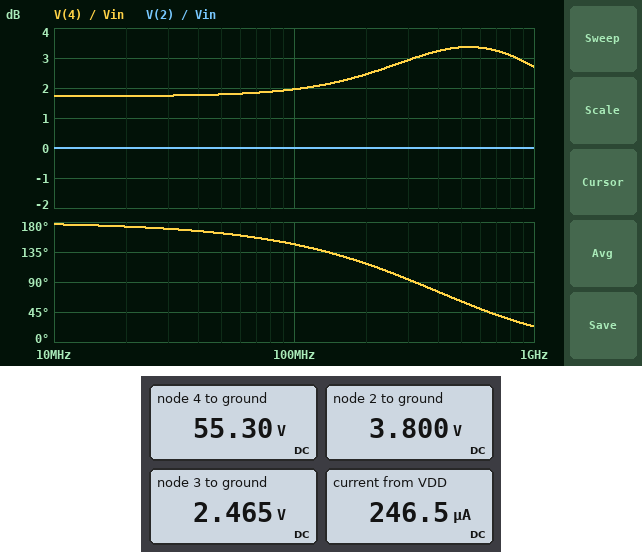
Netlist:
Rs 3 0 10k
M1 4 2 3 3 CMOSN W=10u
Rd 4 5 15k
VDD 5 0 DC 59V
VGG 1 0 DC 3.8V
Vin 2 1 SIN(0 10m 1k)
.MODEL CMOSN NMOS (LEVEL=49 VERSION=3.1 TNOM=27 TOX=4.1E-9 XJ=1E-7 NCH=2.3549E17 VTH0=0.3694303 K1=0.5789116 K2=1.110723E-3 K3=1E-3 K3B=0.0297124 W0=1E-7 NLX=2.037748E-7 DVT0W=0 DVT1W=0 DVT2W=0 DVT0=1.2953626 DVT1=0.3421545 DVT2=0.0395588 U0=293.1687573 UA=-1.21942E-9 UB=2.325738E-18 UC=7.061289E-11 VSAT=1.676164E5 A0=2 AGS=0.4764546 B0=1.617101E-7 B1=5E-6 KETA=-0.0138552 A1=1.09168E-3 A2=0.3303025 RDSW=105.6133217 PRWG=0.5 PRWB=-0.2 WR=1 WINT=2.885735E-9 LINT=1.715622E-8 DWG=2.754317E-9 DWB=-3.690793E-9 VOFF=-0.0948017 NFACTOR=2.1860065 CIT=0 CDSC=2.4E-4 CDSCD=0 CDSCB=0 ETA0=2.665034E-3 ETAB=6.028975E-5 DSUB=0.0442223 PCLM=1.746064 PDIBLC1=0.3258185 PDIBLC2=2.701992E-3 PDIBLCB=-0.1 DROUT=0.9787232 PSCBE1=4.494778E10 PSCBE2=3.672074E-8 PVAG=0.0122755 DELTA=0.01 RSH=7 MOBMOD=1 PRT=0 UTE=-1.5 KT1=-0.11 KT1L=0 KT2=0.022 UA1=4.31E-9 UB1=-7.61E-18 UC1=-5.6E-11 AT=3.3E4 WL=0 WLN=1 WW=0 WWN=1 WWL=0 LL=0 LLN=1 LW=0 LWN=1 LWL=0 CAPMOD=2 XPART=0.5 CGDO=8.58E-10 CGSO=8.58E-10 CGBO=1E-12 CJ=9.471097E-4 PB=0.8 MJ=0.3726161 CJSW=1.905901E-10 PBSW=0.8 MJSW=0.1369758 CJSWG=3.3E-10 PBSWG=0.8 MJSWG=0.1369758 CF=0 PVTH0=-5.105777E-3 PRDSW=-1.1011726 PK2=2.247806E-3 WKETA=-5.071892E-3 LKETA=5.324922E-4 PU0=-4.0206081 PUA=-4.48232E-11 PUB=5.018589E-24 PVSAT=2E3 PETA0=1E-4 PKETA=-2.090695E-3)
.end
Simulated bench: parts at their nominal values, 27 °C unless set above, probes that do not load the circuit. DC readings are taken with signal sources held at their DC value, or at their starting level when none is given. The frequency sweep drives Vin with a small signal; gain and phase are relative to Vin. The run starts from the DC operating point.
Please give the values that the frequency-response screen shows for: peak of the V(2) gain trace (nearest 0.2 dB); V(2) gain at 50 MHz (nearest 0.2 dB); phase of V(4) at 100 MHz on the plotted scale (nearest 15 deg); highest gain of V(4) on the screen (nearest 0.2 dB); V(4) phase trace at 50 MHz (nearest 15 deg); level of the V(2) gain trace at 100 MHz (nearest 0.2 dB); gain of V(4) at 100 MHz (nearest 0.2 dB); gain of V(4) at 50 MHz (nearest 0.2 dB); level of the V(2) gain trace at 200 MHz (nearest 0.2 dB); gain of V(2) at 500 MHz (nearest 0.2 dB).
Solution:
0 dB
0 dB
150 deg
3.4 dB
165 deg
0 dB
2.0 dB
1.8 dB
0 dB
0 dB
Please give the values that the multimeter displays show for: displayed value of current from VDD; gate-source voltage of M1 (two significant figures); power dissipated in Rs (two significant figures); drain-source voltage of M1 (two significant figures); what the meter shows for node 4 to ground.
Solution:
246.5 µA
1.3 V
610 µW
53 V
55.30 V
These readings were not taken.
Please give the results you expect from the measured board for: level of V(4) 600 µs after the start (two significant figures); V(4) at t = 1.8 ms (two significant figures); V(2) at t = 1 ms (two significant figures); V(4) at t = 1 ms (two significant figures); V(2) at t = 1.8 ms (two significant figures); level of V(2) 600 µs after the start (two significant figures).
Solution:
55 V
55 V
3.8 V
55 V
3.8 V
3.8 V
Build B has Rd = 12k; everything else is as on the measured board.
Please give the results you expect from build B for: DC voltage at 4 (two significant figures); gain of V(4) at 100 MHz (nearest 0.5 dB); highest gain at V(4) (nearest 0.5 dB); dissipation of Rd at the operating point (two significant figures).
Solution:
56 V
0 dB
2.0 dB
730 µW
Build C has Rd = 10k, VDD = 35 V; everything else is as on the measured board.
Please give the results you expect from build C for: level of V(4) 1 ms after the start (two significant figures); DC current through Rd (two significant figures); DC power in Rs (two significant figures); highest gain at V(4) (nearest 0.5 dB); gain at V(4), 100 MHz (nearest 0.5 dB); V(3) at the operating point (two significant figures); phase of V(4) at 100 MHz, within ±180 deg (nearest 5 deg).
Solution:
33 V
240 µA
590 µW
0.5 dB
-1.5 dB
2.4 V
150 deg
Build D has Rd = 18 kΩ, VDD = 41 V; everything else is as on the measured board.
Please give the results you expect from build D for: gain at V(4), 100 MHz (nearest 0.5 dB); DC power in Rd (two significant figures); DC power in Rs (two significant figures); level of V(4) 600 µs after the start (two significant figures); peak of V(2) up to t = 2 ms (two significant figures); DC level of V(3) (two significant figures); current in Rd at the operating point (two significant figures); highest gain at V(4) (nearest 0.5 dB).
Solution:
3.5 dB
1.1 mW
590 µW
37 V
3.8 V
2.4 V
240 µA
4.5 dB
